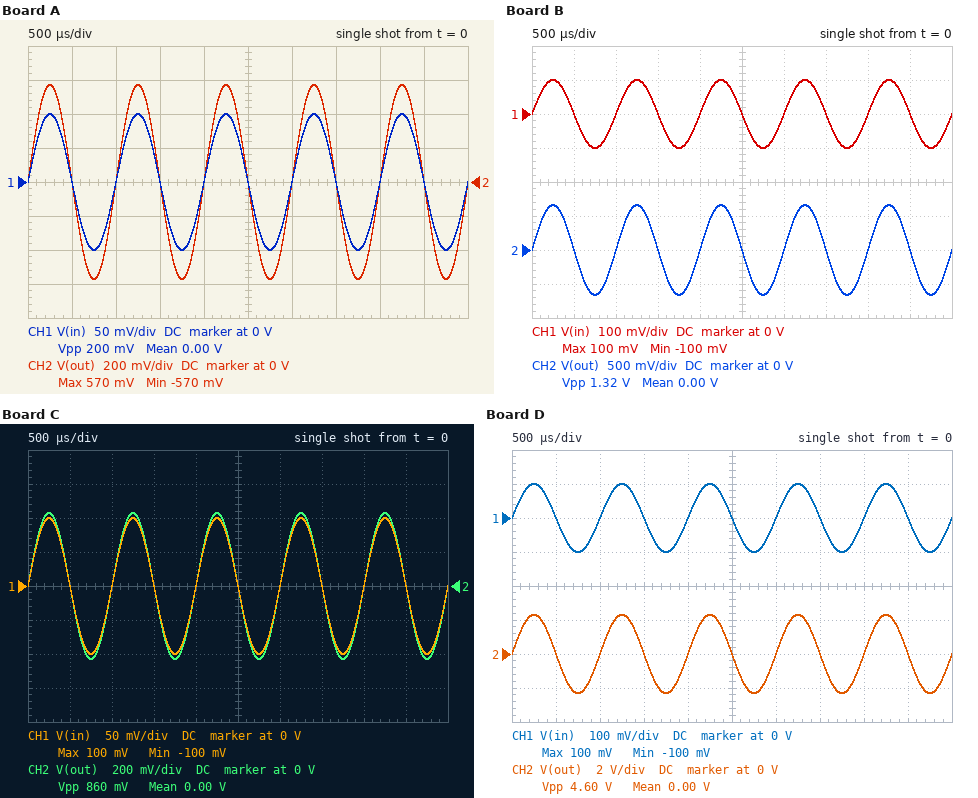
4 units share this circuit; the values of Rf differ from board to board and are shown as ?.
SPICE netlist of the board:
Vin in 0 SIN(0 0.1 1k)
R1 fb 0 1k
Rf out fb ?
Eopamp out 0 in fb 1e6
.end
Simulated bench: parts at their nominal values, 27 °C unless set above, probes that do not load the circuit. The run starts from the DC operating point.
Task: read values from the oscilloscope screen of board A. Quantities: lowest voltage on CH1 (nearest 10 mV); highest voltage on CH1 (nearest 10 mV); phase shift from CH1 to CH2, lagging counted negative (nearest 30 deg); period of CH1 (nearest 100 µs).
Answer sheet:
-100 mV
100 mV
0 deg
1.0 ms
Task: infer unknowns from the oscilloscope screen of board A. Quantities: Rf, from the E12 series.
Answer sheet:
4.7 kΩ
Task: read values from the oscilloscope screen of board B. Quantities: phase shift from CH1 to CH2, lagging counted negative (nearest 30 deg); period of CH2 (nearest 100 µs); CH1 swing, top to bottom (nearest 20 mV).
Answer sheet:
0 deg
1.0 ms
200 mV
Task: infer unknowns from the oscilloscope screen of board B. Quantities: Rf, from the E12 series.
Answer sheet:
5.6 kΩ
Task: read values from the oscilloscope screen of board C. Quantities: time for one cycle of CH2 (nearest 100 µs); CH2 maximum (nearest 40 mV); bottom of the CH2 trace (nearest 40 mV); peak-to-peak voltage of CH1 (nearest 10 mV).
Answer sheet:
1.0 ms
440 mV
-440 mV
200 mV
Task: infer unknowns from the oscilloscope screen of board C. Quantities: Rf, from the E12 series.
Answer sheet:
3.3 kΩ
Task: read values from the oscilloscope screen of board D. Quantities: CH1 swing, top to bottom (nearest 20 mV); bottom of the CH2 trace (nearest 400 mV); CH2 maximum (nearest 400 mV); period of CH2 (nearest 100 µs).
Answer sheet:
200 mV
-2.4 V
2.4 V
1.0 ms
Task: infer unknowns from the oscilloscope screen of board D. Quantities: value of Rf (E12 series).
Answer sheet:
22 kΩ
